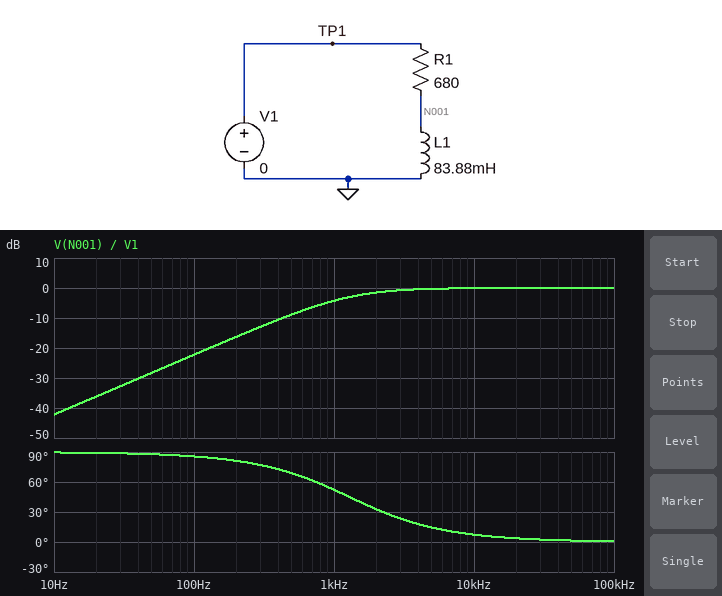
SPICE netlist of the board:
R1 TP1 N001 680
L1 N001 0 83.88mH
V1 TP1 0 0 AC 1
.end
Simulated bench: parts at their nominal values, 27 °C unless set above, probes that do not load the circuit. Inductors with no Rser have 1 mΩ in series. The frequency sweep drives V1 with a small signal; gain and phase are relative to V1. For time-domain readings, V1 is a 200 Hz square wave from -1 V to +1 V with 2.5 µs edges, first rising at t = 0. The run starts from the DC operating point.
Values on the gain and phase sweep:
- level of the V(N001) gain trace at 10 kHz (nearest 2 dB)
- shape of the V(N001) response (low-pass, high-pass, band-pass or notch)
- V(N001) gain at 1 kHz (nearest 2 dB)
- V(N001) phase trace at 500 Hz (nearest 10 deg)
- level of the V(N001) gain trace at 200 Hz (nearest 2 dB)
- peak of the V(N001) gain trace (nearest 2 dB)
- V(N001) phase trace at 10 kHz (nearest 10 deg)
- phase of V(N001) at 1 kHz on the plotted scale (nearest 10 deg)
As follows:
0 dB
high-pass
-4 dB
70 deg
-16 dB
0 dB
10 deg
50 deg
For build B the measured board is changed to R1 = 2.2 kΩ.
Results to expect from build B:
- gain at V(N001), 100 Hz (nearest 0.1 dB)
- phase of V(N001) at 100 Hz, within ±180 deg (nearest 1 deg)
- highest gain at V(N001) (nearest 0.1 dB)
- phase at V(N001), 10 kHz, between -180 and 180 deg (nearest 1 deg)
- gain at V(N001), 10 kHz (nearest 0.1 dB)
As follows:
-32.4 dB
89 deg
0 dB
23 deg
-0.7 dB
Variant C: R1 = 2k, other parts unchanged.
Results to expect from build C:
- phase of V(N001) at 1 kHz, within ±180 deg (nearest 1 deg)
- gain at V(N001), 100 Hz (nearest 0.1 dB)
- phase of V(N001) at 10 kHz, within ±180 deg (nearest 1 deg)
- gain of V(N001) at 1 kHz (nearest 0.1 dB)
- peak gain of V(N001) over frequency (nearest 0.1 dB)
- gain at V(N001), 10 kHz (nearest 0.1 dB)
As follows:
75 deg
-31.6 dB
21 deg
-11.9 dB
0 dB
-0.6 dB
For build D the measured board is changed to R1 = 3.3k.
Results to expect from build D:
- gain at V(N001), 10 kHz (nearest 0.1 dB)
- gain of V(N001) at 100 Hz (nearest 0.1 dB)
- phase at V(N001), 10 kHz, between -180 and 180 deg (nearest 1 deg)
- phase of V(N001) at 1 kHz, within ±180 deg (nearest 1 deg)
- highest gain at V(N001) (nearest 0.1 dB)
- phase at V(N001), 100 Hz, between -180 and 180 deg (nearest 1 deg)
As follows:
-1.4 dB
-35.9 dB
32 deg
81 deg
0 dB
89 deg
